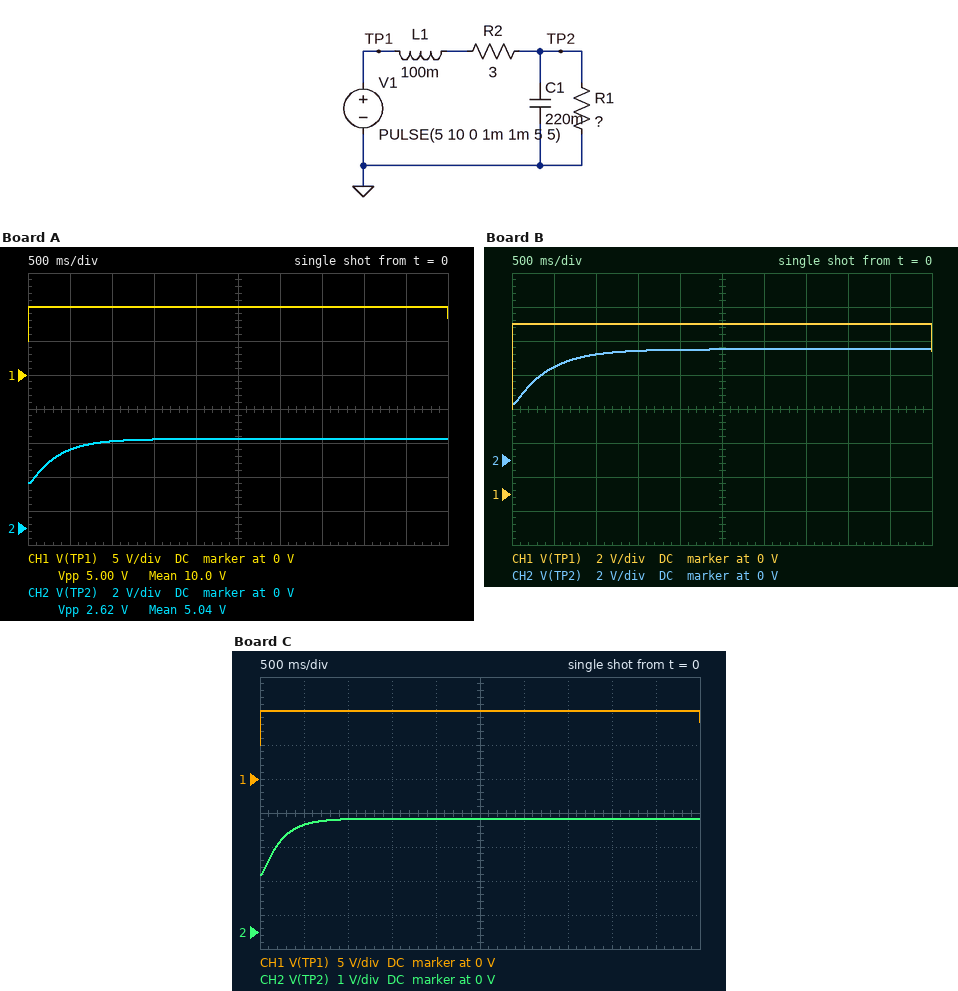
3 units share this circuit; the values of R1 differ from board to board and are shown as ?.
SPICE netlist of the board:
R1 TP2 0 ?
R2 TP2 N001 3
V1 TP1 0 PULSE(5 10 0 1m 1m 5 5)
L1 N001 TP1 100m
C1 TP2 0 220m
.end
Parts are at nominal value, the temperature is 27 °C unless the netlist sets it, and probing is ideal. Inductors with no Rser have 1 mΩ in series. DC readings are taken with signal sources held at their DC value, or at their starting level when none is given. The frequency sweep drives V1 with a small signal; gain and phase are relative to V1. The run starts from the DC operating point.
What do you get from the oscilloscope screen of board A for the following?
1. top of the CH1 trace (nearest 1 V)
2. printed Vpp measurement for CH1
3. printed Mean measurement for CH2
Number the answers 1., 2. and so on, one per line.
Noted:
1. 10 V
2. 5.00 V
3. 5.04 V
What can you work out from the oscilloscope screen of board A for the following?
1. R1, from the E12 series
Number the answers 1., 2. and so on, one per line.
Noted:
1. 3.3 Ω
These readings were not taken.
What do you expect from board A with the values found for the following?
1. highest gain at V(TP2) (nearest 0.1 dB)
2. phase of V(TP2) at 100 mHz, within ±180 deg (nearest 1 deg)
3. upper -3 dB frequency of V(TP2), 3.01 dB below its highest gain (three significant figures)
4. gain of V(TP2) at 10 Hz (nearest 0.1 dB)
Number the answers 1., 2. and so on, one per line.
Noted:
1. -5.6 dB
2. -13 deg
3. 482 mHz
4. -39.6 dB
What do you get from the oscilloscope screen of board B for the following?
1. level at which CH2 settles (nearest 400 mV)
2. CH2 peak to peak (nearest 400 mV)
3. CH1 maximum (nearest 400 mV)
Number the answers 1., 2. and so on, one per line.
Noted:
1. 6.4 V
2. 3.2 V
3. 10.0 V
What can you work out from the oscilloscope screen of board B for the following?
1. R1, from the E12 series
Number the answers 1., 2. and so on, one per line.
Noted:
1. 5.6 Ω
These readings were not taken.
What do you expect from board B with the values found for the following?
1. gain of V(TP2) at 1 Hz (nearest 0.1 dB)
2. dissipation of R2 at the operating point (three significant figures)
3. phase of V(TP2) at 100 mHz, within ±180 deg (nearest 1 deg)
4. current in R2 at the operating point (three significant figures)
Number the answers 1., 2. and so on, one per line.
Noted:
1. -12.7 dB
2. 1.01 W
3. -16 deg
4. 581 mA
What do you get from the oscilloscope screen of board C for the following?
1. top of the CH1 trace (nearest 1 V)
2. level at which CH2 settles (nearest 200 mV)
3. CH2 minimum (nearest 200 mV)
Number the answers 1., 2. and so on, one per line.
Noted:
1. 10 V
2. 3.4 V
3. 1.6 V
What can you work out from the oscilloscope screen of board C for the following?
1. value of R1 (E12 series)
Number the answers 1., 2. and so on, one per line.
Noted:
1. 1.5 Ω
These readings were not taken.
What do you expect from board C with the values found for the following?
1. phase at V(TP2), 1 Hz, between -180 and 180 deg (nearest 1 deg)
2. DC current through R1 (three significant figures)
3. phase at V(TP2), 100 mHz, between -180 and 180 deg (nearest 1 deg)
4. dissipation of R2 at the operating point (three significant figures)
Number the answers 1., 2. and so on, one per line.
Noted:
1. -65 deg
2. 1.11 A
3. -9 deg
4. 3.70 W
